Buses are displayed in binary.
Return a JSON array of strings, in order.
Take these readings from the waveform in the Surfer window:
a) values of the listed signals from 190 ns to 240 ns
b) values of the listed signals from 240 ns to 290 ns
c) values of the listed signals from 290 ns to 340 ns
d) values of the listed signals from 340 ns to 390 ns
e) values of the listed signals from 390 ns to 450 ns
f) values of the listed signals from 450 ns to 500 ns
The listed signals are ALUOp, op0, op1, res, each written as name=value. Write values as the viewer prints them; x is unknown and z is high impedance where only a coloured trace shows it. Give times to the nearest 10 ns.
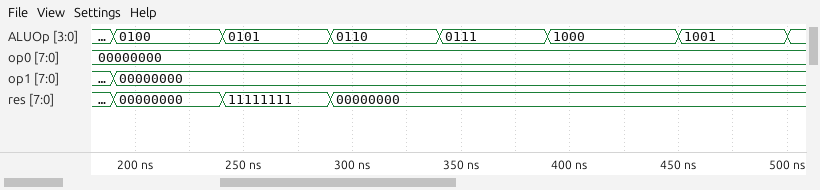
["ALUOp=0100, op0=00000000, op1=00000000, res=00000000", "ALUOp=0101, op0=00000000, op1=00000000, res=11111111", "ALUOp=0110, op0=00000000, op1=00000000, res=00000000", "ALUOp=0111, op0=00000000, op1=00000000, res=00000000", "ALUOp=1000, op0=00000000, op1=00000000, res=00000000", "ALUOp=1001, op0=00000000, op1=00000000, res=00000000"]
